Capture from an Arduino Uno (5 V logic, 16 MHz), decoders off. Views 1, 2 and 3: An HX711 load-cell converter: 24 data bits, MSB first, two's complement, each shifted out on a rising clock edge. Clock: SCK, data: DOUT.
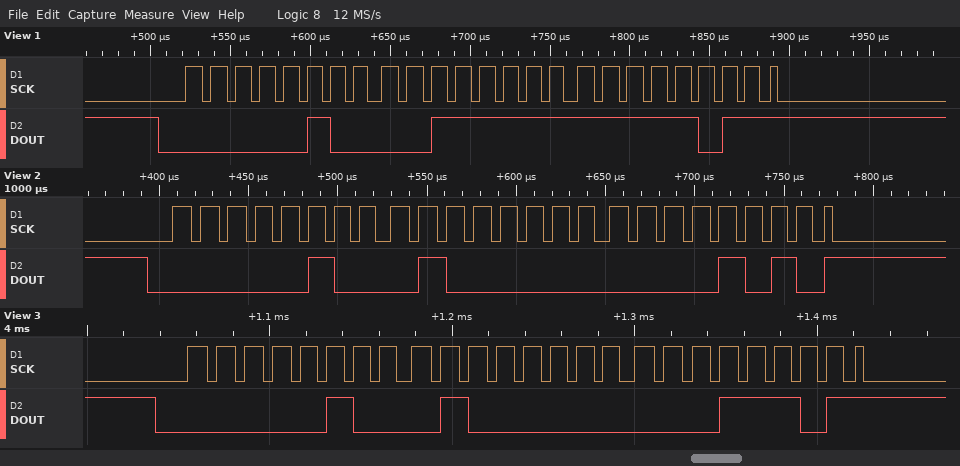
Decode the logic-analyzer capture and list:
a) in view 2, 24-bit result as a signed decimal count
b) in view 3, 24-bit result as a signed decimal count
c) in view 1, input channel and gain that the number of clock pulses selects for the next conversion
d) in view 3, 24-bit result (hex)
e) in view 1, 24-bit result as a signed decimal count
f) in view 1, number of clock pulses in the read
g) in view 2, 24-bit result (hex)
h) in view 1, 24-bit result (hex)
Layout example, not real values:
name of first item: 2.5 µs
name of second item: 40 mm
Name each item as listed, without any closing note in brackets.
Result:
in view 2, 24-bit result as a signed decimal count: 278538
in view 3, 24-bit result as a signed decimal count: 278557
in view 1, input channel and gain that the number of clock pulses selects for the next conversion: channel A, gain 128
in view 3, 24-bit result: 0x04401D
in view 1, 24-bit result as a signed decimal count: 278523
in view 1, number of clock pulses in the read: 25
in view 2, 24-bit result: 0x04400A
in view 1, 24-bit result: 0x043FFB
